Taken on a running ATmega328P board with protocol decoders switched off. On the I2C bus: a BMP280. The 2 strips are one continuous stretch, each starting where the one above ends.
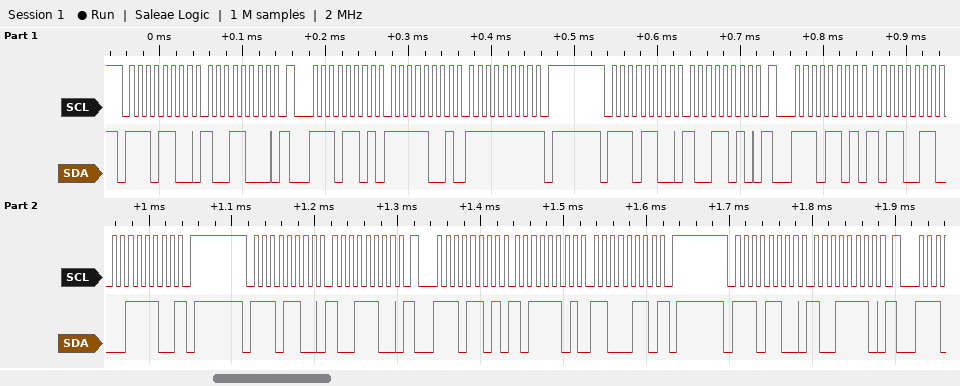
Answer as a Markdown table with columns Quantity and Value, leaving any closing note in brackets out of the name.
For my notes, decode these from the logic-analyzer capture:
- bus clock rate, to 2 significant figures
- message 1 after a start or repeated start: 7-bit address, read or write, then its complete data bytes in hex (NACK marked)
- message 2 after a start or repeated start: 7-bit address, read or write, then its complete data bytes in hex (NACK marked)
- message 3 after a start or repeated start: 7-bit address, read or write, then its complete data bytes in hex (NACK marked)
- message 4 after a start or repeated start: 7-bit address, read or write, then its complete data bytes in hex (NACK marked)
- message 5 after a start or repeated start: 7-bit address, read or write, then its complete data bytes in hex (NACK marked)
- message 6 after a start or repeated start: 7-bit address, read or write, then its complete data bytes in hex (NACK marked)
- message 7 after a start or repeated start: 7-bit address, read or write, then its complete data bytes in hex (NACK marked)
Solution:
| Quantity | Value |
|---|---|
| bus clock rate, to 2 significant figures | 100 kHz |
| message 1 after a start or repeated start: 7-bit address, read or write, then its complete data bytes in hex | 0x76 write: 98 |
| message 2 after a start or repeated start: 7-bit address, read or write, then its complete data bytes in hex | 0x76 read: F9 FF NACK |
| message 3 after a start or repeated start: 7-bit address, read or write, then its complete data bytes in hex | 0x76 write: 9A |
| message 4 after a start or repeated start: 7-bit address, read or write, then its complete data bytes in hex | 0x76 read: B3 3C NACK |
| message 5 after a start or repeated start: 7-bit address, read or write, then its complete data bytes in hex | 0x76 write: 9C |
| message 6 after a start or repeated start: 7-bit address, read or write, then its complete data bytes in hex | 0x76 read: BD C6 NACK |
| message 7 after a start or repeated start: 7-bit address, read or write, then its complete data bytes in hex | 0x76 write: 9E |
